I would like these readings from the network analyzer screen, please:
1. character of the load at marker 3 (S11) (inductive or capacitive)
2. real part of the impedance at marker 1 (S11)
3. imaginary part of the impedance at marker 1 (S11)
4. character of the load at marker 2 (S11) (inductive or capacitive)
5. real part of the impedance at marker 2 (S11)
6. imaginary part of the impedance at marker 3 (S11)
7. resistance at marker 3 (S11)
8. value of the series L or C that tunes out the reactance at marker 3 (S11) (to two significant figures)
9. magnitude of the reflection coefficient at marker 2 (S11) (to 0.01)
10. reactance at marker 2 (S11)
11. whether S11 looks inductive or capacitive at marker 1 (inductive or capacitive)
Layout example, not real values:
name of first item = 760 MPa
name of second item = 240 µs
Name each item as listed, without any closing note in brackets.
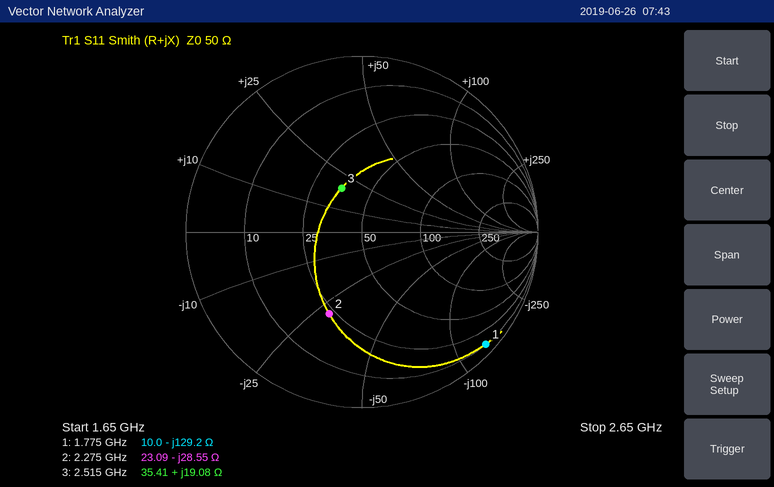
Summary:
character of the load at marker 3 (S11) = inductive
real part of the impedance at marker 1 = 10.0 Ω
imaginary part of the impedance at marker 1 = -129.2 Ω
character of the load at marker 2 (S11) = capacitive
real part of the impedance at marker 2 = 23.09 Ω
imaginary part of the impedance at marker 3 = +19.08 Ω
resistance at marker 3 = 35.41 Ω
value of the series L or C that tunes out the reactance at marker 3 (S11) = 3.3 pF
magnitude of the reflection coefficient at marker 2 (S11) = 0.50
reactance at marker 2 = -28.55 Ω
whether S11 looks inductive or capacitive at marker 1 = capacitive
